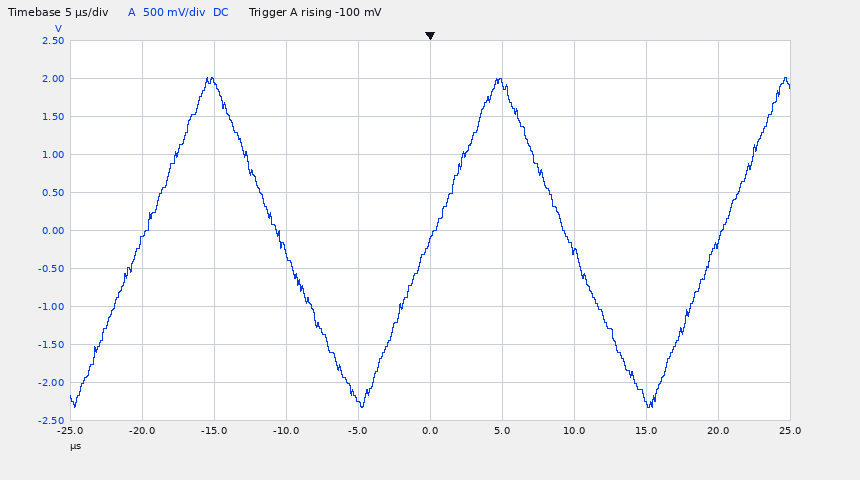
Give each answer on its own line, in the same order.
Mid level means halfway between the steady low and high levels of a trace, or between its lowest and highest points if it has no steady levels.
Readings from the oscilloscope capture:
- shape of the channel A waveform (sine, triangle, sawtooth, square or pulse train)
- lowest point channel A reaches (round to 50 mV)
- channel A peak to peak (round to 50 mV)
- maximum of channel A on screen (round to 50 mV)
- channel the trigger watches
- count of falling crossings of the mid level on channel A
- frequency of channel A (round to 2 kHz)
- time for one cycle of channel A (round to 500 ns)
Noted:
triangle
-2.35 V
4.35 V
2.00 V
channel A
2
50 kHz
20.0 µs
